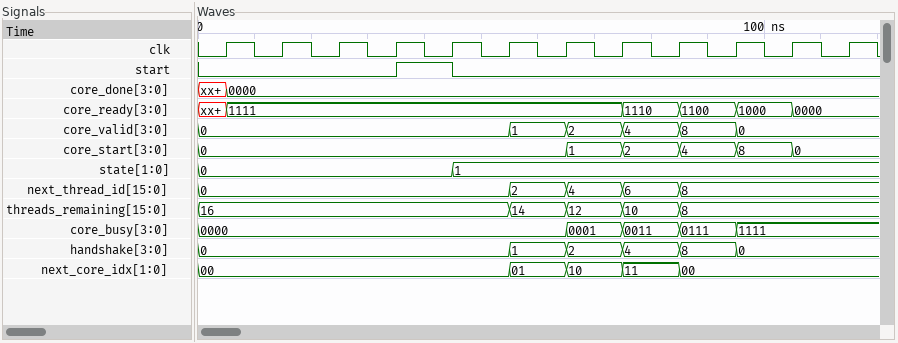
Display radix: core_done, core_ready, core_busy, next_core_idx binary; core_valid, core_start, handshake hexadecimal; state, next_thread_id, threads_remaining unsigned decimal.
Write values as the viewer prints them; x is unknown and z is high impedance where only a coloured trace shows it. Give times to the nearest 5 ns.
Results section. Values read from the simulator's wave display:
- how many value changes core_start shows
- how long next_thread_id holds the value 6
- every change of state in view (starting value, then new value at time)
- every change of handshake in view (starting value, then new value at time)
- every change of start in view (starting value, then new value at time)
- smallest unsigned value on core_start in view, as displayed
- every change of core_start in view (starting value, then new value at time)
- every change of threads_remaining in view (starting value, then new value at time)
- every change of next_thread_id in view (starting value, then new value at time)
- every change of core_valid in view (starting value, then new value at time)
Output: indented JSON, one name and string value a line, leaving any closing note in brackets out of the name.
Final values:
{
  "how many value changes core_start shows": "5",
  "how long next_thread_id holds the value 6": "10 ns",
  "every change of state in view": "0, 1 at 45 ns",
  "every change of handshake in view": "0, 1 at 55 ns, 2 at 65 ns, 4 at 75 ns, 8 at 85 ns, 0 at 95 ns",
  "every change of start in view": "0, 1 at 35 ns, 0 at 45 ns",
  "smallest unsigned value on core_start in view, as displayed": "0",
  "every change of core_start in view": "0, 1 at 65 ns, 2 at 75 ns, 4 at 85 ns, 8 at 95 ns, 0 at 105 ns",
  "every change of threads_remaining in view": "16, 14 at 55 ns, 12 at 65 ns, 10 at 75 ns, 8 at 85 ns",
  "every change of next_thread_id in view": "0, 2 at 55 ns, 4 at 65 ns, 6 at 75 ns, 8 at 85 ns",
  "every change of core_valid in view": "0, 1 at 55 ns, 2 at 65 ns, 4 at 75 ns, 8 at 85 ns, 0 at 95 ns"
}
